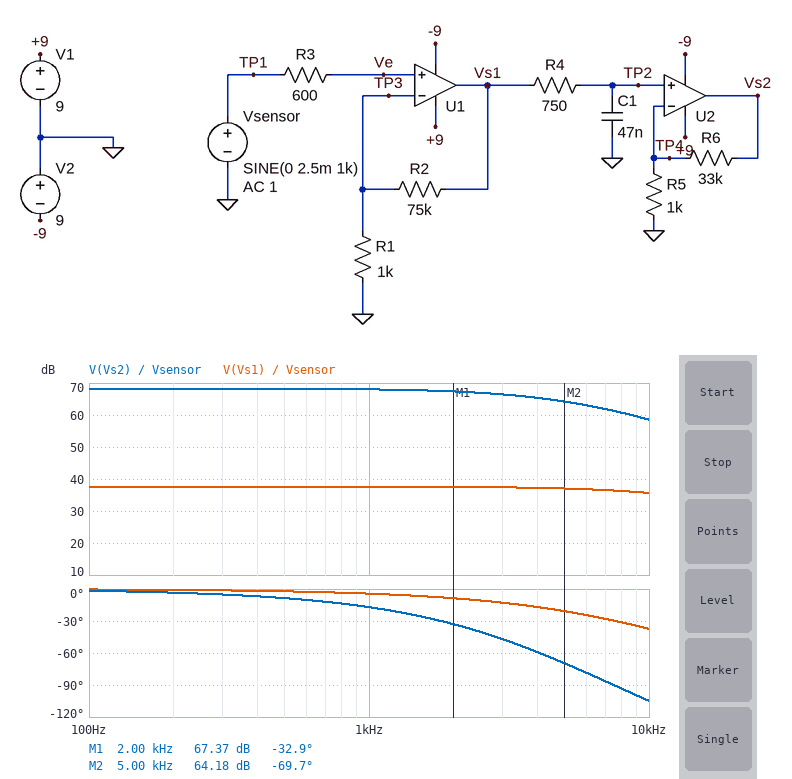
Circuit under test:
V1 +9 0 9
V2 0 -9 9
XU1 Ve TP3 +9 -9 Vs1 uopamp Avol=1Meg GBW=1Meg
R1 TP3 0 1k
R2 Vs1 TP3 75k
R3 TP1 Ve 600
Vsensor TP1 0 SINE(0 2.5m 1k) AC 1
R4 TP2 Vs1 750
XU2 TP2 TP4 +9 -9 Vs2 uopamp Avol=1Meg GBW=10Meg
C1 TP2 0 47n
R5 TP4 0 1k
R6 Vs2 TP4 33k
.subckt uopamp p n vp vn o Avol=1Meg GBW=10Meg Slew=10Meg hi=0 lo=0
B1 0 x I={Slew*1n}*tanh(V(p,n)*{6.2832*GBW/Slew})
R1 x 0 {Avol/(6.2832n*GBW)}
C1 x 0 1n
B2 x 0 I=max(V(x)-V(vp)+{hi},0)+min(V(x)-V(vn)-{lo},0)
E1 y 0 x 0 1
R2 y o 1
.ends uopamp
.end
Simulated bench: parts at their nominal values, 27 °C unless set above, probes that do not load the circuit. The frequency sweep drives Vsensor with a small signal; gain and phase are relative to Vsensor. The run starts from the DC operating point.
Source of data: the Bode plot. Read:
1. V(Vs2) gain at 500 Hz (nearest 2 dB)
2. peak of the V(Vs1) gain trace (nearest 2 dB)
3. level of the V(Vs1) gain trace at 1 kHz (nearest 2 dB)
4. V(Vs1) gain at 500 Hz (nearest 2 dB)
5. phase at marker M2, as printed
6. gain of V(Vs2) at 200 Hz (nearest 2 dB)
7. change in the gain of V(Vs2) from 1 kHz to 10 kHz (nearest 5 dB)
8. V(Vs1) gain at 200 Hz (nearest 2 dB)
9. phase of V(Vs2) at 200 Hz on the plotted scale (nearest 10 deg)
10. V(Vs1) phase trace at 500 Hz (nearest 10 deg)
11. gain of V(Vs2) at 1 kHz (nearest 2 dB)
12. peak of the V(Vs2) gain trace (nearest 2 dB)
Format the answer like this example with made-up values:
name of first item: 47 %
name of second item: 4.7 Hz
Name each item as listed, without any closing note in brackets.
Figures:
V(Vs2) gain at 500 Hz: 68 dB
peak of the V(Vs1) gain trace: 38 dB
level of the V(Vs1) gain trace at 1 kHz: 38 dB
V(Vs1) gain at 500 Hz: 38 dB
phase at marker M2, as printed: -69.7 deg
gain of V(Vs2) at 200 Hz: 68 dB
change in the gain of V(Vs2) from 1 kHz to 10 kHz: -10 dB
V(Vs1) gain at 200 Hz: 38 dB
phase of V(Vs2) at 200 Hz on the plotted scale: 0 deg
V(Vs1) phase trace at 500 Hz: 0 deg
gain of V(Vs2) at 1 kHz: 68 dB
peak of the V(Vs2) gain trace: 68 dB
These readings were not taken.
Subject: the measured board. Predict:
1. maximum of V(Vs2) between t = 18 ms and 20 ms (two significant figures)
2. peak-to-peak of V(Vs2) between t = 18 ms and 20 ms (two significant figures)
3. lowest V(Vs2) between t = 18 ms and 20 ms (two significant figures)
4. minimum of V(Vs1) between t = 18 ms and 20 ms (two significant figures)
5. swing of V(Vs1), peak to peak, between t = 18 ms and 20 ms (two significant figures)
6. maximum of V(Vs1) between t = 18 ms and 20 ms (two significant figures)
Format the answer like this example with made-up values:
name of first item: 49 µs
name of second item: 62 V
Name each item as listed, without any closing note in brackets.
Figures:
maximum of V(Vs2) between t = 18 ms and 20 ms: 6.3 V
peak-to-peak of V(Vs2) between t = 18 ms and 20 ms: 13 V
lowest V(Vs2) between t = 18 ms and 20 ms: -6.3 V
minimum of V(Vs1) between t = 18 ms and 20 ms: -190 mV
swing of V(Vs1), peak to peak, between t = 18 ms and 20 ms: 380 mV
maximum of V(Vs1) between t = 18 ms and 20 ms: 190 mV
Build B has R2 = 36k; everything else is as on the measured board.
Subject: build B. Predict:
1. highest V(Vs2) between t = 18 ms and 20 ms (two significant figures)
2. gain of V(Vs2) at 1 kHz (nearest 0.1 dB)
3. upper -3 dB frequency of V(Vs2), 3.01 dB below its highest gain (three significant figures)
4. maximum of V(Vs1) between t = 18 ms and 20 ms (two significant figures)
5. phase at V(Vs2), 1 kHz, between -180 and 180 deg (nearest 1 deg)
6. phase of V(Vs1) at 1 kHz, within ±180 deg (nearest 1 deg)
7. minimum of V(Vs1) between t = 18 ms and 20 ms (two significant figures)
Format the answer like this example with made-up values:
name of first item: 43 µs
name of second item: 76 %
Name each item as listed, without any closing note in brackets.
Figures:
highest V(Vs2) between t = 18 ms and 20 ms: 3.1 V
gain of V(Vs2) at 1 kHz: 61.8 dB
upper -3 dB frequency of V(Vs2), 3.01 dB below its highest gain: 4.40 kHz
maximum of V(Vs1) between t = 18 ms and 20 ms: 92 mV
phase at V(Vs2), 1 kHz, between -180 and 180 deg: -15 deg
phase of V(Vs1) at 1 kHz, within ±180 deg: -2 deg
minimum of V(Vs1) between t = 18 ms and 20 ms: -92 mV
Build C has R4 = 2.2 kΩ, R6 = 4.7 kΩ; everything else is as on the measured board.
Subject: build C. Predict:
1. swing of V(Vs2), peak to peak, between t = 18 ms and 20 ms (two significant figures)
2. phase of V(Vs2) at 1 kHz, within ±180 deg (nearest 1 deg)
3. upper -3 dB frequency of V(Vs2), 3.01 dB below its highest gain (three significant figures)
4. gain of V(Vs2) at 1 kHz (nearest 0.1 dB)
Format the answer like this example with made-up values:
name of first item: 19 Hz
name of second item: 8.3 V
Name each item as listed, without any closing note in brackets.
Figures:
swing of V(Vs2), peak to peak, between t = 18 ms and 20 ms: 1.8 V
phase of V(Vs2) at 1 kHz, within ±180 deg: -37 deg
upper -3 dB frequency of V(Vs2), 3.01 dB below its highest gain: 1.52 kHz
gain of V(Vs2) at 1 kHz: 51.2 dB
